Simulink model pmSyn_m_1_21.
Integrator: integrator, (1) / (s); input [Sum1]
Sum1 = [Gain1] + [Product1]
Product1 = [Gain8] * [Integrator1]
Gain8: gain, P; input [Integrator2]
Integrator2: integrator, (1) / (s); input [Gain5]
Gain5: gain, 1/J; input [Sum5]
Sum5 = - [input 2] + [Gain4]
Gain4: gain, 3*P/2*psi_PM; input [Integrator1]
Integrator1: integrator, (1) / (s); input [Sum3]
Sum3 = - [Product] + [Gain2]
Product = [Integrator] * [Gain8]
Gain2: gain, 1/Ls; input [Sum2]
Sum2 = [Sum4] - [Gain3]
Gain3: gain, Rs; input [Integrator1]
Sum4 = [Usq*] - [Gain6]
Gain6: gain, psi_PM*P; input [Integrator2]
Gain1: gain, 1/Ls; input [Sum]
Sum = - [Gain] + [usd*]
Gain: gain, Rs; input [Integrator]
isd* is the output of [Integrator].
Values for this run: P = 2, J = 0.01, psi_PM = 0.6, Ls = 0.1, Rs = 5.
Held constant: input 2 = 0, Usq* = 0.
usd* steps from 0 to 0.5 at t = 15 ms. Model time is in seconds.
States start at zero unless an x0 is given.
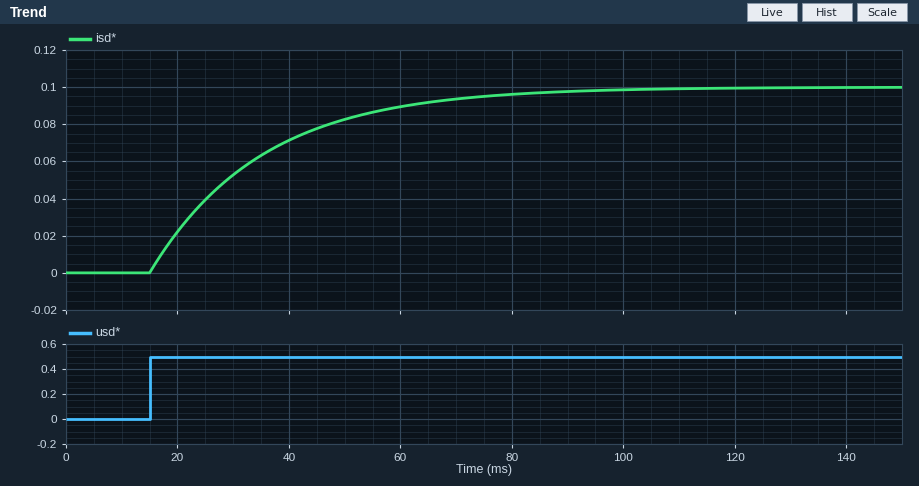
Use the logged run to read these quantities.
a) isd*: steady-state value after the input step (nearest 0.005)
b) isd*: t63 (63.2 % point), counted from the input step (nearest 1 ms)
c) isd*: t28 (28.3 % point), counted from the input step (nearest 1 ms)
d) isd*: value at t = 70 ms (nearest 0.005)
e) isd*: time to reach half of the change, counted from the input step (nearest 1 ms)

0.100
20 ms
7 ms
0.095
14 ms
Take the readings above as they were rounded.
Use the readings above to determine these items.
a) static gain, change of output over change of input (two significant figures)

0.20
